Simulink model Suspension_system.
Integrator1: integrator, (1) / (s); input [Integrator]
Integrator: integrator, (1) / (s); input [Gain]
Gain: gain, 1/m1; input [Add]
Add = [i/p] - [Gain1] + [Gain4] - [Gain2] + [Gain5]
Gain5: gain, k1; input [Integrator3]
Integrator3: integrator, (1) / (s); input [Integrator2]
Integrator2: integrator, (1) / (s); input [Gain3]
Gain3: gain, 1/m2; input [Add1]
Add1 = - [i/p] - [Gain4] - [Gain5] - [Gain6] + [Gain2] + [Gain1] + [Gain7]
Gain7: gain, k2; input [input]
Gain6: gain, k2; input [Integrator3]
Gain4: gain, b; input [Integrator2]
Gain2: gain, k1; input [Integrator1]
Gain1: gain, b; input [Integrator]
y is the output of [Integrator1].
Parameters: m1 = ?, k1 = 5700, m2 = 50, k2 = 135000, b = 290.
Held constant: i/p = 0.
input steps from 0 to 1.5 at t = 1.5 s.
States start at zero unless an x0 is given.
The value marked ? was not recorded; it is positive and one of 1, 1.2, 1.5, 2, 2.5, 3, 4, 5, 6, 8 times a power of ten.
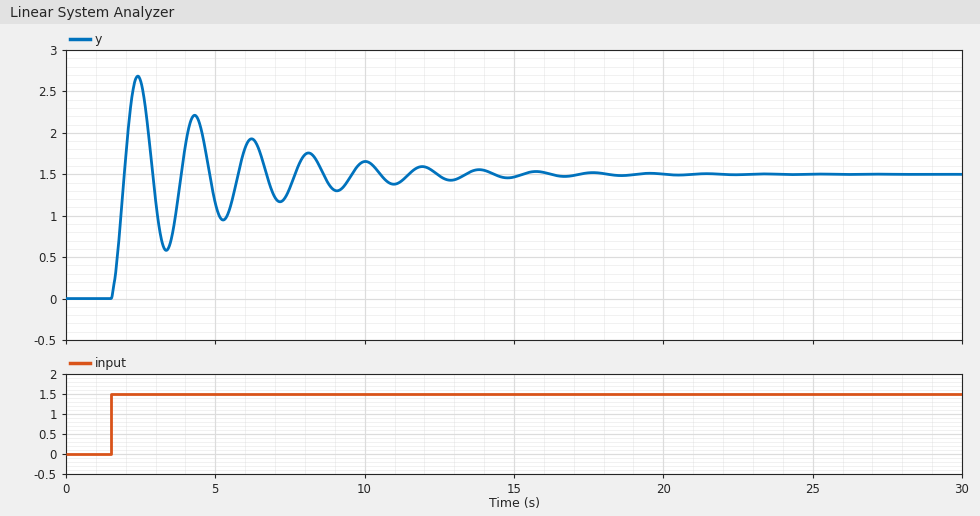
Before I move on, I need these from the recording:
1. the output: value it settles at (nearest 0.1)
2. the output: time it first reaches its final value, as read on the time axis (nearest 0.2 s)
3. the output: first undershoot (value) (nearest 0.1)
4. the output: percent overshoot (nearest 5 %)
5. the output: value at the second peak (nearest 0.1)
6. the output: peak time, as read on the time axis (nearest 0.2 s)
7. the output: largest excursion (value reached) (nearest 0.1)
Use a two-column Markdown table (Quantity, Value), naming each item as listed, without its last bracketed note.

| Quantity | Value |
|---|---|
| the output: value it settles at | 1.5 |
| the output: time it first reaches its final value, as read on the time axis | 2.0 s |
| the output: first undershoot (value) | 0.6 |
| the output: percent overshoot | 80 % |
| the output: value at the second peak | 2.2 |
| the output: peak time, as read on the time axis | 2.4 s |
| the output: largest excursion (value reached) | 2.7 |
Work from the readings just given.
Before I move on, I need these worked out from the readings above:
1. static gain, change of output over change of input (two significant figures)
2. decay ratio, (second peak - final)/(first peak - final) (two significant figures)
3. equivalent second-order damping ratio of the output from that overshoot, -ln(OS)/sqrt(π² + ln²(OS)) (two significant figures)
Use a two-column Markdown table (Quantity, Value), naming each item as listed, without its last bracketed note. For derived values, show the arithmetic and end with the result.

| Quantity | Value |
|---|---|
| static gain, change of output over change of input | (1.5 - 0) / (1.5 - 0) = 1.0 |
| decay ratio, (second peak - final)/(first peak - final) | (2.2 - 1.5) / (2.7 - 1.5) = 0.58 |
| equivalent second-order damping ratio of the output from that overshoot, -ln(OS)/sqrt(π² + ln²(OS)) | ln(0.8) = -0.223; 0.223 / sqrt(9.870 + 0.050) = 0.071 |
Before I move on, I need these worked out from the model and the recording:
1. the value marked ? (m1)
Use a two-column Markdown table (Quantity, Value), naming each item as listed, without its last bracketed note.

| Quantity | Value |
|---|---|
| the value marked ? | 500 |
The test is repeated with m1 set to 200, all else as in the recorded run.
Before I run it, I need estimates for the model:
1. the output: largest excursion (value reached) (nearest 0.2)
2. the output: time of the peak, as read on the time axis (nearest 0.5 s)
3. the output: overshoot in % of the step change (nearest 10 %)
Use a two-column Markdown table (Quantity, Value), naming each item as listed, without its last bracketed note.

| Quantity | Value |
|---|---|
| the output: largest excursion (value reached) | 2.6 |
| the output: time of the peak, as read on the time axis | 2.0 s |
| the output: overshoot in % of the step change | 70 % |
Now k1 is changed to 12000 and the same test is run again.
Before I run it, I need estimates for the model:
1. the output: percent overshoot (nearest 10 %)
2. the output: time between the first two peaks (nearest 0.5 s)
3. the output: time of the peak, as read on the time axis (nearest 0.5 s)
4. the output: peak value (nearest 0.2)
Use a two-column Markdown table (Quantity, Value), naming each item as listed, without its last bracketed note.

| Quantity | Value |
|---|---|
| the output: percent overshoot | 90 % |
| the output: time between the first two peaks | 1.5 s |
| the output: time of the peak, as read on the time axis | 2.0 s |
| the output: peak value | 2.8 |
